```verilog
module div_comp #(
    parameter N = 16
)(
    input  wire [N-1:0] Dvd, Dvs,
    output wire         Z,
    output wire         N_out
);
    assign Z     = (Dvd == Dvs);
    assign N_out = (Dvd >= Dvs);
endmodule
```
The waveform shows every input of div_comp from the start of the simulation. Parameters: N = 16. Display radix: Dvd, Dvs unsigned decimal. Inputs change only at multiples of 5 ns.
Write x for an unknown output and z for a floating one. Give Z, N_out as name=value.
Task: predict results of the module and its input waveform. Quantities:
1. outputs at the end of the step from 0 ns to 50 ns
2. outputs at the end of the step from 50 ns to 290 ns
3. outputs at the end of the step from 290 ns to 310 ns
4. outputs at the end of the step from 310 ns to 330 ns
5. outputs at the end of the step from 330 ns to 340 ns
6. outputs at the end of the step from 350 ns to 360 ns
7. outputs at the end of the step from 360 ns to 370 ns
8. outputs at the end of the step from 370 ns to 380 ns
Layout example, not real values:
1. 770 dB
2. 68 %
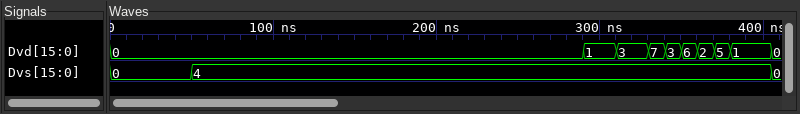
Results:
1. Z=1, N_out=1
2. Z=0, N_out=0
3. Z=0, N_out=0
4. Z=0, N_out=0
5. Z=0, N_out=1
6. Z=0, N_out=1
7. Z=0, N_out=0
8. Z=0, N_out=1
